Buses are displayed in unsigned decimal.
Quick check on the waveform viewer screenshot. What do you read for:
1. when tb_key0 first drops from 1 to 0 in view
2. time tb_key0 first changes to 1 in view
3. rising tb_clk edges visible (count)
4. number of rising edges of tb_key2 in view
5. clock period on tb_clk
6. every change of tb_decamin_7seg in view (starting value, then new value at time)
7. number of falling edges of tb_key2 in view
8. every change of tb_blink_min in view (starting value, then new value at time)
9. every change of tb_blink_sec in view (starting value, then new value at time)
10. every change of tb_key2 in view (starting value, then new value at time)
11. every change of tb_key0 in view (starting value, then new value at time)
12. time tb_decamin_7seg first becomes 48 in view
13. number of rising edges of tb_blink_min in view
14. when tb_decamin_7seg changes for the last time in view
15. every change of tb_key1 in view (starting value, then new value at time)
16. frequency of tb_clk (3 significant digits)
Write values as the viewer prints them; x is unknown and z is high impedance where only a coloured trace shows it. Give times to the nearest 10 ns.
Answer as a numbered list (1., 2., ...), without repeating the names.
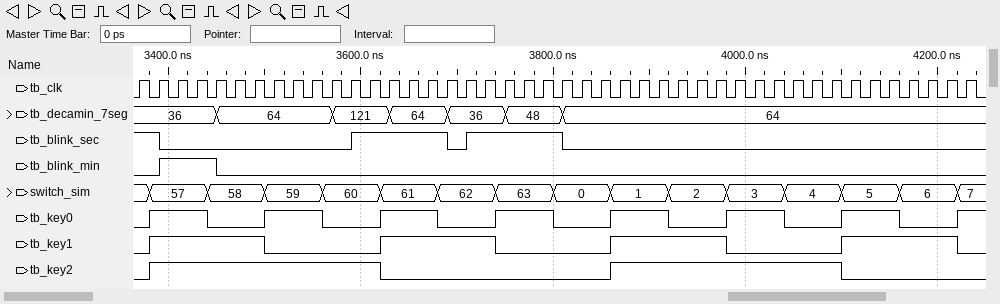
1. 3440 ns
2. 3380 ns
3. 44
4. 2
5. 20 ns
6. 36, 64 at 3450 ns, 121 at 3570 ns, 64 at 3630 ns, 36 at 3690 ns, 48 at 3750 ns, 64 at 3810 ns
7. 2
8. 0, 1 at 3390 ns, 0 at 3450 ns
9. 1, 0 at 3390 ns, 1 at 3590 ns, 0 at 3690 ns, 1 at 3710 ns, 0 at 3810 ns
10. 0, 1 at 3380 ns, 0 at 3620 ns, 1 at 3860 ns, 0 at 4100 ns
11. 0, 1 at 3380 ns, 0 at 3440 ns, 1 at 3500 ns, 0 at 3560 ns, 1 at 3620 ns, 0 at 3680 ns, 1 at 3740 ns, 0 at 3800 ns, 1 at 3860 ns, 0 at 3920 ns, 1 at 3980 ns, 0 at 4040 ns, 1 at 4100 ns, 0 at 4160 ns, 1 at 4220 ns
12. 3750 ns
13. 1
14. 3810 ns
15. 0, 1 at 3380 ns, 0 at 3500 ns, 1 at 3620 ns, 0 at 3740 ns, 1 at 3860 ns, 0 at 3980 ns, 1 at 4100 ns, 0 at 4220 ns
16. 50.0 MHz
